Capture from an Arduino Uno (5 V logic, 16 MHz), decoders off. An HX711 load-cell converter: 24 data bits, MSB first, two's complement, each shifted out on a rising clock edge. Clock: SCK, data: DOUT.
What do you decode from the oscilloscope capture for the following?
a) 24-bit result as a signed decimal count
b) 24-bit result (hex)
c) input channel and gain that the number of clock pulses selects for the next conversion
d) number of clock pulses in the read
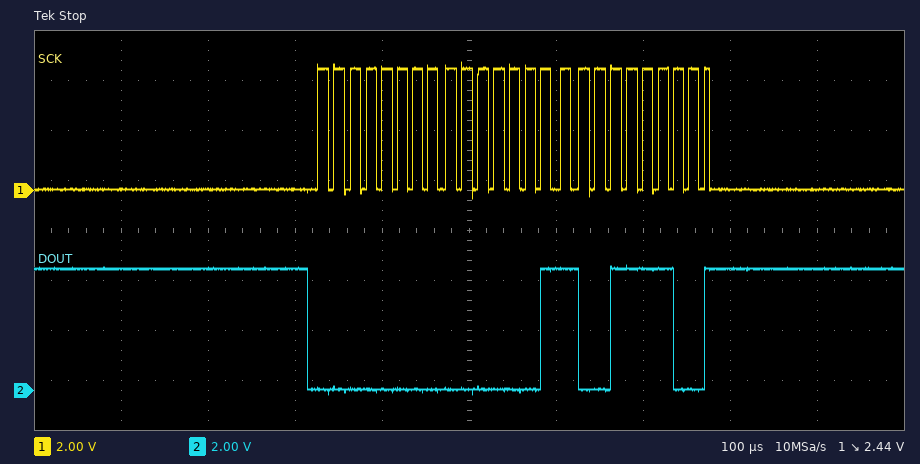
828
0x00033C
channel A, gain 128
25
